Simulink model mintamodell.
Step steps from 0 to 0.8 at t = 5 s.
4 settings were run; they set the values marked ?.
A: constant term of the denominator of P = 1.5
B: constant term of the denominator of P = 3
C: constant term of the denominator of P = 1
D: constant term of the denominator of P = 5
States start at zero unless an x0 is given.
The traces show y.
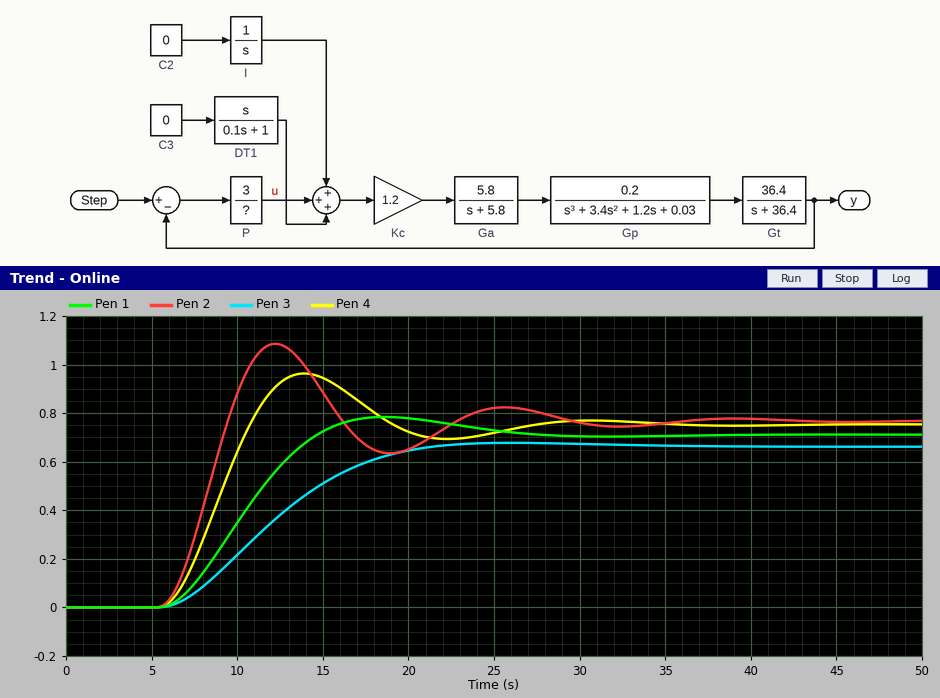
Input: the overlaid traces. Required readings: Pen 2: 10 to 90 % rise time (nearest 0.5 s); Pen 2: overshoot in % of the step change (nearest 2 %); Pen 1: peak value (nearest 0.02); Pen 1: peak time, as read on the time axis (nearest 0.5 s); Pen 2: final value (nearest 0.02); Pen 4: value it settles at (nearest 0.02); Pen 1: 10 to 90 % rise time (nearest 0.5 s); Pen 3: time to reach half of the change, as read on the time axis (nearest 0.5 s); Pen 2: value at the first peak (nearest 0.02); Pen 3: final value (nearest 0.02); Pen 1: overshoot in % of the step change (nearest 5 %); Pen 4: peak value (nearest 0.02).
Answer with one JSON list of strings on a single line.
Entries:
["2.5 s", "42 %", "0.78", "18.5 s", "0.76", "0.76", "6.0 s", "11.5 s", "1.08", "0.66", "10 %", "0.96"]
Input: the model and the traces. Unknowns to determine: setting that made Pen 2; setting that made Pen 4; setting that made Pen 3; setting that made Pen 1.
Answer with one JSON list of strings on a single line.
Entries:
["C", "A", "D", "B"]
